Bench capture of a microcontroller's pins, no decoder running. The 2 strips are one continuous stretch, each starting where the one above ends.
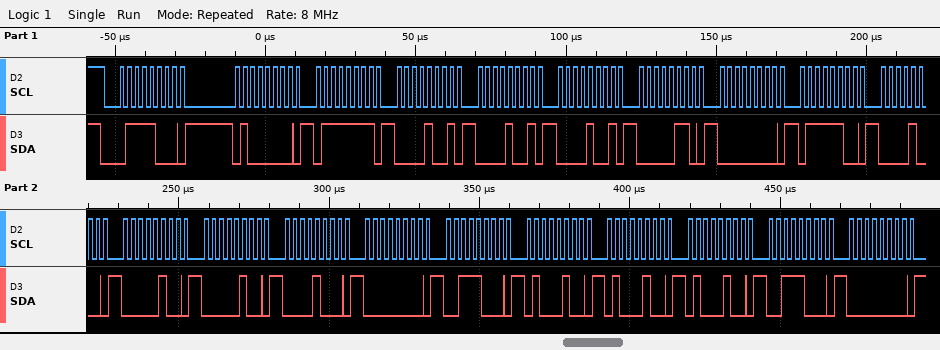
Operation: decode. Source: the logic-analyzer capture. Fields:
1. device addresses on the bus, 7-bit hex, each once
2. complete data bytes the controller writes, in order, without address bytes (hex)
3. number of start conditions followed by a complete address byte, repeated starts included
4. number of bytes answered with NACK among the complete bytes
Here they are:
0x3C
40 7F 09 09 09 06 00 7C 08 04 04 08 00 38 44 44 44 38 00
1
0
